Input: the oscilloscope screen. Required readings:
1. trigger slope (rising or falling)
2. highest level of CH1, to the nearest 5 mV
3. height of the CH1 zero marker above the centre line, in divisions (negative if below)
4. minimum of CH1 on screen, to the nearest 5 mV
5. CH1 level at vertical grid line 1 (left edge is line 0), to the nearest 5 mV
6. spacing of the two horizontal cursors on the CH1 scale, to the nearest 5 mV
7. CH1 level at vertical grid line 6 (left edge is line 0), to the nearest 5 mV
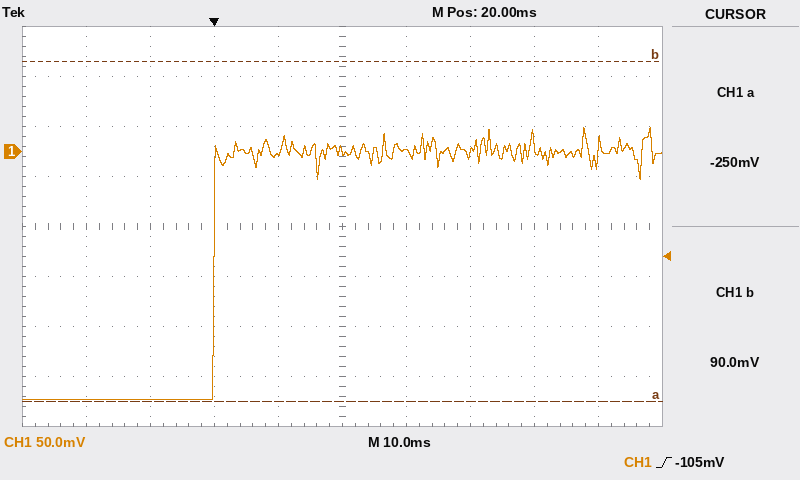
rising
25 mV
+1.5 div
-250 mV
-250 mV
340 mV
0 mV
